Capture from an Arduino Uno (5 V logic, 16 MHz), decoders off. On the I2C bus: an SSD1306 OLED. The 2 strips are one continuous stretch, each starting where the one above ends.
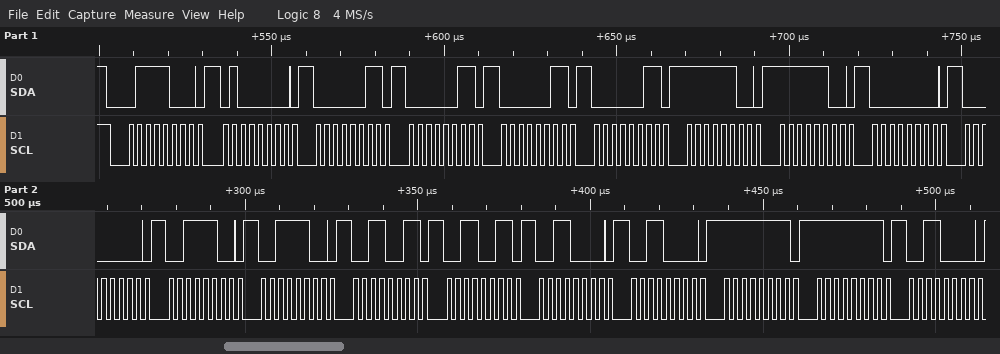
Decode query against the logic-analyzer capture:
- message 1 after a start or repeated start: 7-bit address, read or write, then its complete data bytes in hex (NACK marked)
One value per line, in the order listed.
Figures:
0x3C write: 40 03 03 03 03 FC FC 00 00 3C 3C 33 33 30 30 FF FF 30
